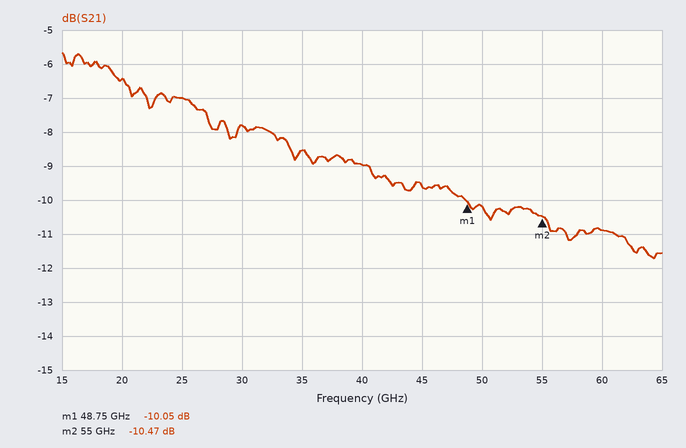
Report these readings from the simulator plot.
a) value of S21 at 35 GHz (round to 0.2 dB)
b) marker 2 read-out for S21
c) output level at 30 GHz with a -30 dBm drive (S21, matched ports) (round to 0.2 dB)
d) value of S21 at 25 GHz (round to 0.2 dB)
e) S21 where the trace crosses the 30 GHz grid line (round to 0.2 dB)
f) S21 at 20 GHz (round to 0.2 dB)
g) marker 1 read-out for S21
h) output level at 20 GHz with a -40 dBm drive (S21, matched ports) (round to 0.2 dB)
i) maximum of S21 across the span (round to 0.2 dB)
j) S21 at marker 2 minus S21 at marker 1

-8.6 dB
-10.47 dB
-37.8 dBm
-7.0 dB
-7.8 dB
-6.4 dB
-10.05 dB
-46.4 dBm
-5.6 dB
-0.42 dB
